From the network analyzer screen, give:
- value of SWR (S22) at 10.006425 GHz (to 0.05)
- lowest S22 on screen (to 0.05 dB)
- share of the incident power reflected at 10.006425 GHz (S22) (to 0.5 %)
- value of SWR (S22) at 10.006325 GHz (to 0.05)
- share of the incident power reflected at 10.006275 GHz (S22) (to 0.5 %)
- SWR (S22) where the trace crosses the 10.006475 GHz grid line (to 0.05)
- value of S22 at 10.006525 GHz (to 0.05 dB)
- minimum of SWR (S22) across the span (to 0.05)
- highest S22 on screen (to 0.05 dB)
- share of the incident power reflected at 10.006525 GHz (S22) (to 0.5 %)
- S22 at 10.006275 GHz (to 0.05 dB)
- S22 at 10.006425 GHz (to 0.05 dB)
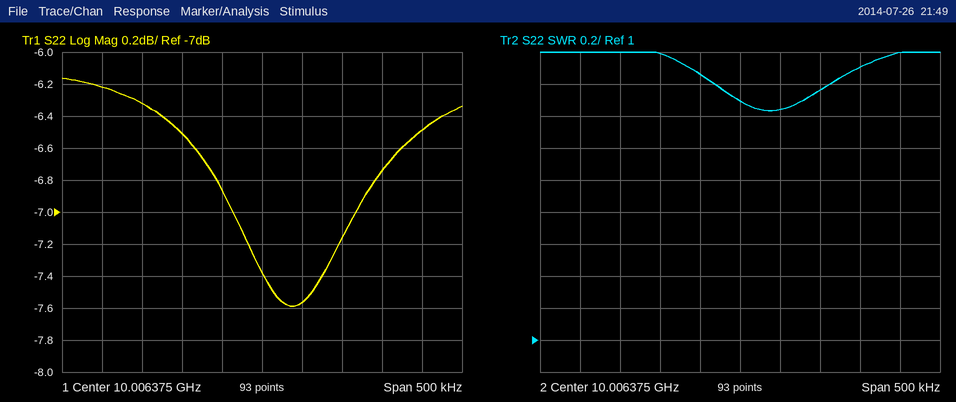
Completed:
2.45
-7.60 dB
17.5 %
2.65
22.5 %
2.55
-6.75 dB
2.45
-6.15 dB
21.0 %
-6.50 dB
-7.55 dB
